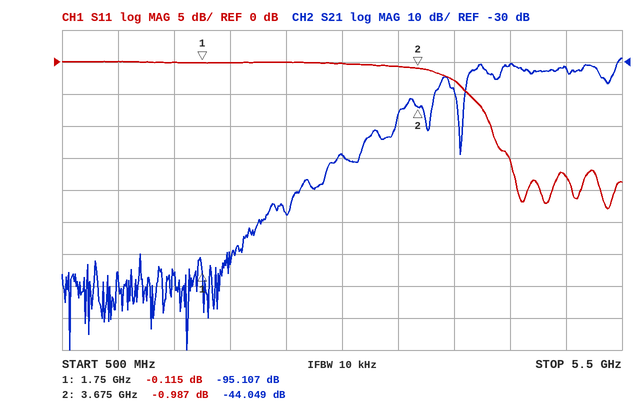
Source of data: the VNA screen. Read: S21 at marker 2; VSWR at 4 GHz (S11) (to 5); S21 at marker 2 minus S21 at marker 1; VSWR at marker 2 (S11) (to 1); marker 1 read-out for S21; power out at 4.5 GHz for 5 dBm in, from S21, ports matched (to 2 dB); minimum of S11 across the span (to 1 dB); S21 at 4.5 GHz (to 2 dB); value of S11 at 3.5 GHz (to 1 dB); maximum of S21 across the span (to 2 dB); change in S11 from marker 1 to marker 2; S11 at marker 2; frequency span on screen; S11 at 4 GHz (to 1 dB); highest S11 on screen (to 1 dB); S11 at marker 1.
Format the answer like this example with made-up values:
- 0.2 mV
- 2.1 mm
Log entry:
- -44.049 dB
- 5
- 51.058 dB
- 18
- -95.107 dB
- -26 dBm
- -23 dB
- -30 dB
- -1 dB
- -28 dB
- -0.872 dB
- -0.987 dB
- 5 GHz
- -3 dB
- 0 dB
- -0.115 dB
